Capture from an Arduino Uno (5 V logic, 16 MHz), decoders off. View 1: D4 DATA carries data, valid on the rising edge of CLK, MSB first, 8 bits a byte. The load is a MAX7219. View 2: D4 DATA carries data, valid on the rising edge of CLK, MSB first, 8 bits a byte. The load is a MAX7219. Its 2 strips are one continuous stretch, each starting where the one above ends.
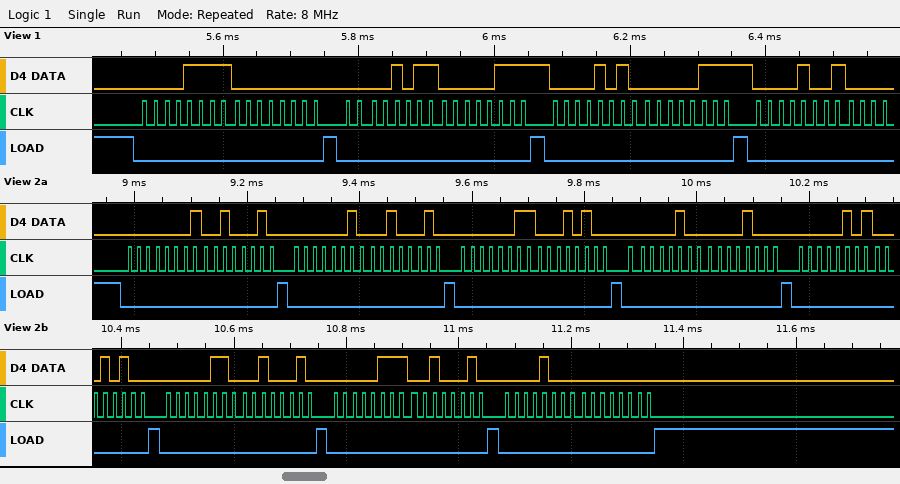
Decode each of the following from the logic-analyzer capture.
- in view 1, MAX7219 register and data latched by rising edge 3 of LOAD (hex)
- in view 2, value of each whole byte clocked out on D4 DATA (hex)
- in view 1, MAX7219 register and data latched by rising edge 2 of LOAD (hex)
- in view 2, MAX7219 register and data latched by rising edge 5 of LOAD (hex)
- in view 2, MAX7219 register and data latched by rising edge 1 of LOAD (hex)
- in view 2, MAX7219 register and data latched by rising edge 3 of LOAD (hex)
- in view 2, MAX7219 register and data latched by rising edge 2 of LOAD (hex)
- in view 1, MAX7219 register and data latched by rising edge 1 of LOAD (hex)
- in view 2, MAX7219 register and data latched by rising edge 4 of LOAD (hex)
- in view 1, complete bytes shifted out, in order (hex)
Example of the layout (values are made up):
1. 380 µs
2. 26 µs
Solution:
1. register 0xA, data 0x07
2. 0x01 0x22 0x02 0x22 0x03 0x14 0x04 0x08 0x05 0x14 0x06 0x22 0x07 0x22 0x08 0x00
3. register 0xB, data 0x07
4. register 0x5, data 0x14
5. register 0x1, data 0x22
6. register 0x3, data 0x14
7. register 0x2, data 0x22
8. register 0xF, data 0x00
9. register 0x4, data 0x08
10. 0x0F 0x00 0x0B 0x07 0x0A 0x07 0x09
